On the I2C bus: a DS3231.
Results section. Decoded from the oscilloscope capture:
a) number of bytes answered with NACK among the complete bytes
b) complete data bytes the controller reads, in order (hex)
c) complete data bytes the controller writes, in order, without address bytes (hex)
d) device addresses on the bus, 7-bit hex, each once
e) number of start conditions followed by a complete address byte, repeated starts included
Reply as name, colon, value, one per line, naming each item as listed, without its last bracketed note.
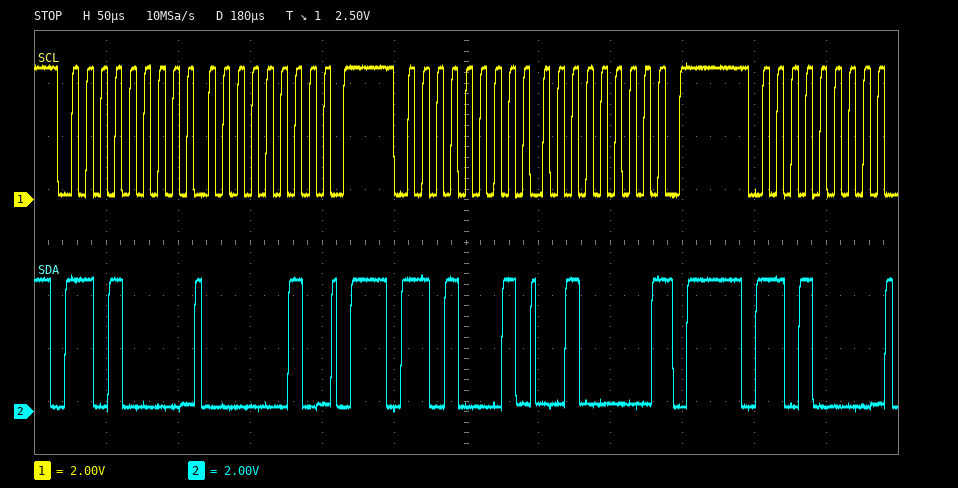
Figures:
number of bytes answered with NACK among the complete bytes: 1
complete data bytes the controller reads, in order: 20
complete data bytes the controller writes, in order, without address bytes: 02
device addresses on the bus, 7-bit hex, each once: 0x68
number of start conditions followed by a complete address byte, repeated starts included: 3
